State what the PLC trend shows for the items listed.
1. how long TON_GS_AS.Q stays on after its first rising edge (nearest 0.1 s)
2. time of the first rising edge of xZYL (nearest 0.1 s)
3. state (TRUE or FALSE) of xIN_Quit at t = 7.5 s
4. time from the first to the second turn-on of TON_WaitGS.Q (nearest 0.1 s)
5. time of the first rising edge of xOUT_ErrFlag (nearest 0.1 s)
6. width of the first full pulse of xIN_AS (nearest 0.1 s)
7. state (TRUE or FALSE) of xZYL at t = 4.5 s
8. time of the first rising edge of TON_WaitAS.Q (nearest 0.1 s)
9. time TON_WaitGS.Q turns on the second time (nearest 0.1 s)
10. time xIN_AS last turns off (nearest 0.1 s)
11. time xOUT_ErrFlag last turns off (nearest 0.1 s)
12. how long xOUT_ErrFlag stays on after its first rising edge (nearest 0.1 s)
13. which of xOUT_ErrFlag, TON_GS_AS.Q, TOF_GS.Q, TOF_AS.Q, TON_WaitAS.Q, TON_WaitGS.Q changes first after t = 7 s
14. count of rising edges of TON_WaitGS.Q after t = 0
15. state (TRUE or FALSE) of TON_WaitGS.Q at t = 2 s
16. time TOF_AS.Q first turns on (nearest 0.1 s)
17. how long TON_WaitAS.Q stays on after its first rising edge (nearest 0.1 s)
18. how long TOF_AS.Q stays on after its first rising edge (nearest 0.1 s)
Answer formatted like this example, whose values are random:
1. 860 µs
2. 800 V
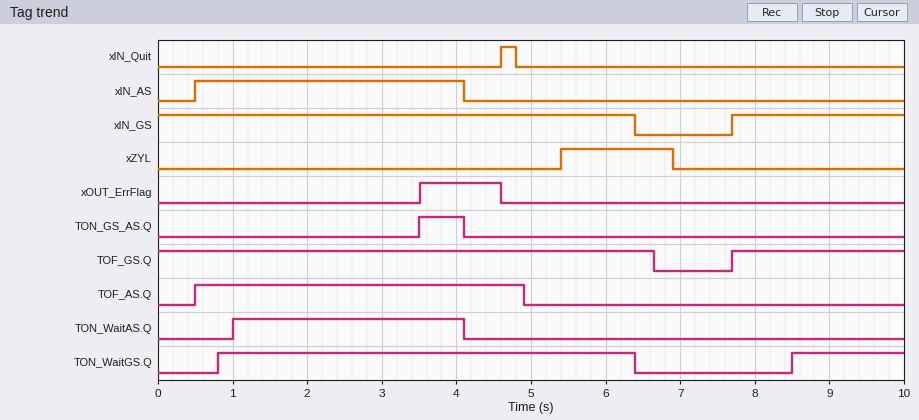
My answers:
1. 0.6 s
2. 5.4 s
3. FALSE
4. 7.7 s
5. 3.5 s
6. 3.6 s
7. FALSE
8. 1.0 s
9. 8.5 s
10. 4.1 s
11. 4.6 s
12. 1.1 s
13. TOF_GS.Q
14. 2
15. TRUE
16. 0.5 s
17. 3.1 s
18. 4.4 s
